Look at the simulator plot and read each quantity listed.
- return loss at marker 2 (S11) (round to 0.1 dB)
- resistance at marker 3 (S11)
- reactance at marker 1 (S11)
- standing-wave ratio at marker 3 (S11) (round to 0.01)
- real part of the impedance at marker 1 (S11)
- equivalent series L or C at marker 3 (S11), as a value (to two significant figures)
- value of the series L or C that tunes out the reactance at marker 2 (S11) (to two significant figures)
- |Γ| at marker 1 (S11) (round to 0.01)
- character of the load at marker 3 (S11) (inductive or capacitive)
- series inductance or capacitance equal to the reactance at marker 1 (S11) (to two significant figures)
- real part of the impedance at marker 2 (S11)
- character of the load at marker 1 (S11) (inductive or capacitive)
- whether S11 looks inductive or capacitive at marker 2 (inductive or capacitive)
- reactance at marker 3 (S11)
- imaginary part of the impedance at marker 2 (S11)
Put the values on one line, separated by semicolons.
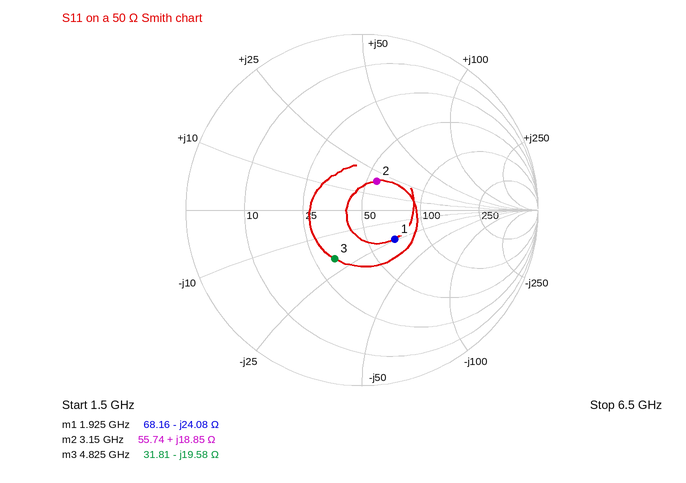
14.7 dB; 31.81 Ω; -24.08 Ω; 1.93; 68.16 Ω; 1.7 pF; 2.7 pF; 0.25; capacitive; 3.4 pF; 55.74 Ω; capacitive; inductive; -19.58 Ω; +18.85 Ω
